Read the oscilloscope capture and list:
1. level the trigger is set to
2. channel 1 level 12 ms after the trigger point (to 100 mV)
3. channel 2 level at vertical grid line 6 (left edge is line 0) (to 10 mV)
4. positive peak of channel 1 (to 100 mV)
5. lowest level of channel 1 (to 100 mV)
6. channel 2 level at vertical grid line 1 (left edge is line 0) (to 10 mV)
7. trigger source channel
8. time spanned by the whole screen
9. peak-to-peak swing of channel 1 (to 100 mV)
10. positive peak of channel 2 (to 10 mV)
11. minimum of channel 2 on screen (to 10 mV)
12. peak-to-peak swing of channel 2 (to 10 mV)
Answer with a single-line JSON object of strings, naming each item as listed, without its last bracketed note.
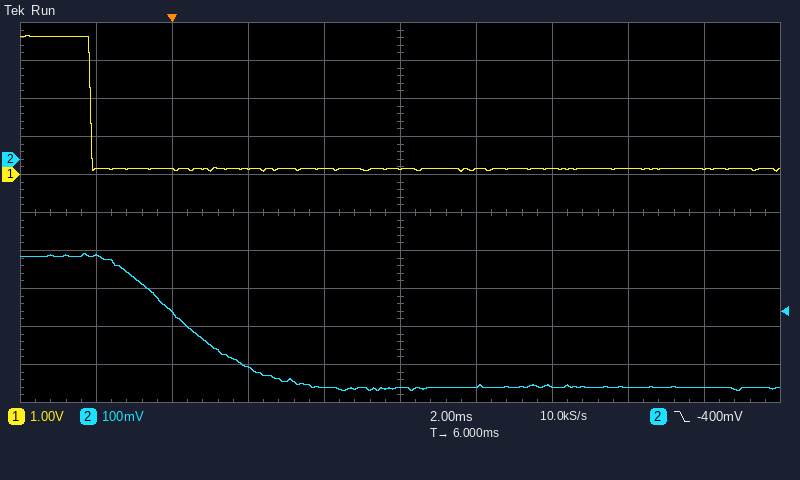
{"level the trigger is set to": "-400 mV", "channel 1 level 12 ms after the trigger point": "200 mV", "channel 2 level at vertical grid line 6 (left edge is line 0)": "-600 mV", "positive peak of channel 1": "3.7 V", "lowest level of channel 1": "100 mV", "channel 2 level at vertical grid line 1 (left edge is line 0)": "-250 mV", "trigger source channel": "channel 2", "time spanned by the whole screen": "20 ms", "peak-to-peak swing of channel 1": "3.6 V", "positive peak of channel 2": "-250 mV", "minimum of channel 2 on screen": "-610 mV", "peak-to-peak swing of channel 2": "360 mV"}
